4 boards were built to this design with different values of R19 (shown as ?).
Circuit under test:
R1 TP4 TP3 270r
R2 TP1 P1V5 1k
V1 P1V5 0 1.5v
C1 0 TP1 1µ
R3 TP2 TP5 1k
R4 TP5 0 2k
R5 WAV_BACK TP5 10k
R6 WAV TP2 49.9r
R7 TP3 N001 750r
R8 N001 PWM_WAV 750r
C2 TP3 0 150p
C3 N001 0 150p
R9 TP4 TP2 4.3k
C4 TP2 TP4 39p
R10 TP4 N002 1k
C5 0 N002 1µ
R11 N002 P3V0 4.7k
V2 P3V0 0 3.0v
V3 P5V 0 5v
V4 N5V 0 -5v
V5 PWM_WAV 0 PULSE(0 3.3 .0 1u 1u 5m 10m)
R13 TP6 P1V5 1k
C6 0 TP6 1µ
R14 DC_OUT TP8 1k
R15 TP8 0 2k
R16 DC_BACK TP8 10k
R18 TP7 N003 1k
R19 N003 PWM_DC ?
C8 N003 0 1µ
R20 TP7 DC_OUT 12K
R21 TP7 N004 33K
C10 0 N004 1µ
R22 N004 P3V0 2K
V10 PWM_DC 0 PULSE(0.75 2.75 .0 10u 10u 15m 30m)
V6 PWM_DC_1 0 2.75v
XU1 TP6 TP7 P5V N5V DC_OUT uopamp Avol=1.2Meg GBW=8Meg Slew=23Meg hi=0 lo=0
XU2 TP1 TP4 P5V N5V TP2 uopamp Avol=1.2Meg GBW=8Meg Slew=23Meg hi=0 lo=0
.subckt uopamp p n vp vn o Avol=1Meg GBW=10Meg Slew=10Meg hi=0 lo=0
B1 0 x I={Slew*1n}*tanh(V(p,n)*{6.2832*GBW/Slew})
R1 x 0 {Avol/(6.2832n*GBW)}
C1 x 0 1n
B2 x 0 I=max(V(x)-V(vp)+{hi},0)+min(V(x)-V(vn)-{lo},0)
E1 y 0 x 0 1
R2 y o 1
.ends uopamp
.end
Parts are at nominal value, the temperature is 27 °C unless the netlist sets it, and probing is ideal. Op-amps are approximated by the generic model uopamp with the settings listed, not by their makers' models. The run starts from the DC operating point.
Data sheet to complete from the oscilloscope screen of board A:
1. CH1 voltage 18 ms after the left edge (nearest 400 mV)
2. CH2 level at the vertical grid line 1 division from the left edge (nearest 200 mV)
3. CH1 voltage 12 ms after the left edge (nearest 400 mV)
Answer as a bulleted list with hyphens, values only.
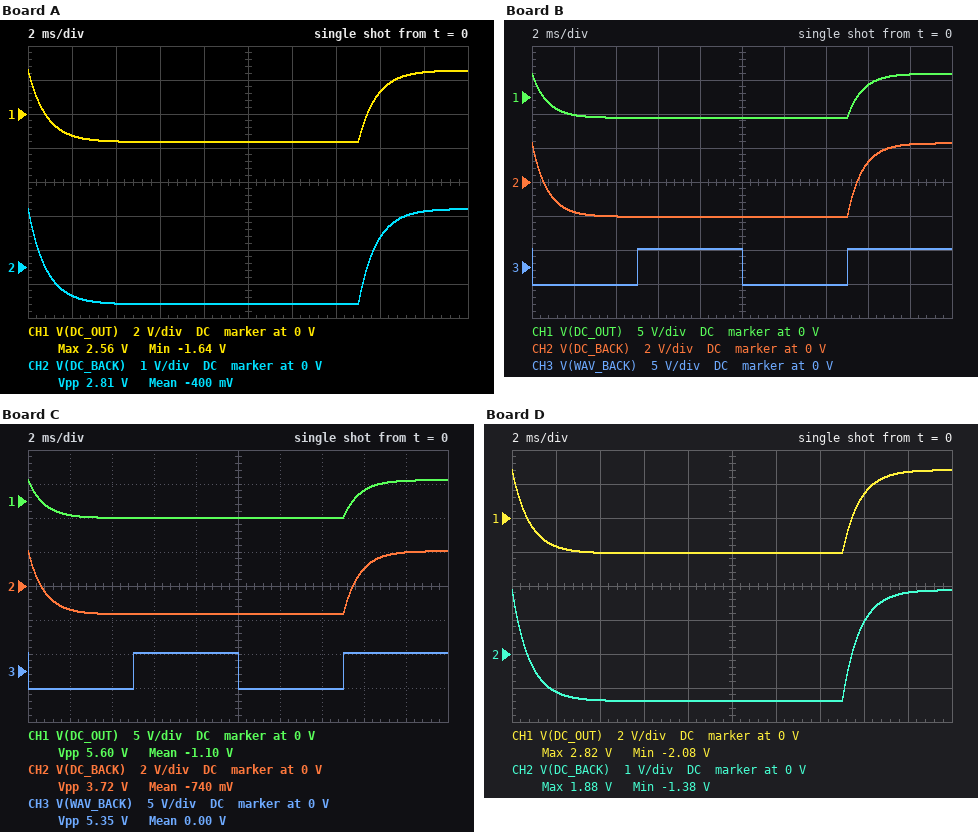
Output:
- 2.4 V
- -800 mV
- -1.6 V
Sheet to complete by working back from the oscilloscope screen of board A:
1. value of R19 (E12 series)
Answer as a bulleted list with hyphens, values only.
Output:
- 4.7 kΩ
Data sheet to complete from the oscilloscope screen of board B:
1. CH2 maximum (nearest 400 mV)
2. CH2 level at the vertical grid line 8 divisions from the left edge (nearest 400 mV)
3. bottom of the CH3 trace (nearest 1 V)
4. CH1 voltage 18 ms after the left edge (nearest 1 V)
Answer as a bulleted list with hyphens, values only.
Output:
- 2.4 V
- 1.2 V
- -3 V
- 3 V
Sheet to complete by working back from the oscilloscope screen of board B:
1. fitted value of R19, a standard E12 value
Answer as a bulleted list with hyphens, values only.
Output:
- 2.7 kΩ
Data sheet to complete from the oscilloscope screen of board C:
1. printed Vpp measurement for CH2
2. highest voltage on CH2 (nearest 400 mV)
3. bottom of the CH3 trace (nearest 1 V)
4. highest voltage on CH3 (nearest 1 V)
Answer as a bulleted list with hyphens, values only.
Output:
- 3.72 V
- 2.0 V
- -3 V
- 3 V
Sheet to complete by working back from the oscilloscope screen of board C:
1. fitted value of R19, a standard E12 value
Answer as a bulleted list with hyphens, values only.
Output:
- 3.3 kΩ
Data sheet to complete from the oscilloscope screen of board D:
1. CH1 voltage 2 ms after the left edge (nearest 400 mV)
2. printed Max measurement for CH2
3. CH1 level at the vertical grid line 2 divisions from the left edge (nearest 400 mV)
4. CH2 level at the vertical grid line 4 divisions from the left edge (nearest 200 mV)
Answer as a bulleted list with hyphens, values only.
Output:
- -1.6 V
- 1.88 V
- -2.0 V
- -1.4 V
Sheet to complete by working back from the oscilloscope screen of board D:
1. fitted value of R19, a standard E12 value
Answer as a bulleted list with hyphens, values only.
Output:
- 3.9 kΩ
